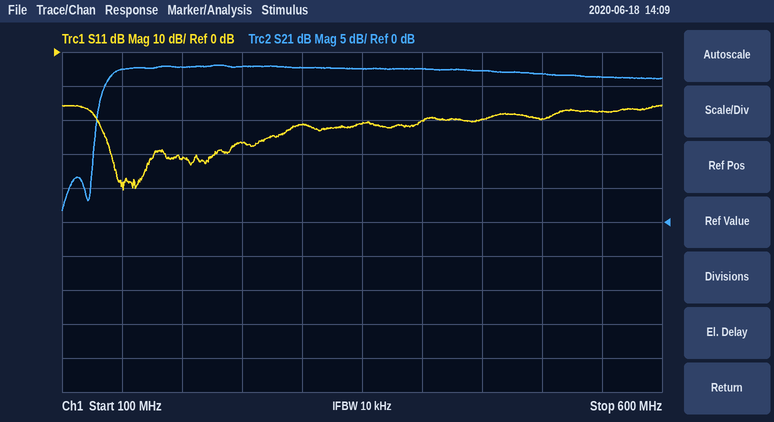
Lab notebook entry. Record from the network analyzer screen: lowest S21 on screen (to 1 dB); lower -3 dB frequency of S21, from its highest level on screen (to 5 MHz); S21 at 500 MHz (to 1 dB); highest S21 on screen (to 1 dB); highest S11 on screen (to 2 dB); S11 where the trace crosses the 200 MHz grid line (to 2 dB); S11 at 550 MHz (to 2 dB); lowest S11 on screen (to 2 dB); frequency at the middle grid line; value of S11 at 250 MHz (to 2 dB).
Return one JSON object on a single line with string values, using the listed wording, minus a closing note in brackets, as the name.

{"lowest S21 on screen": "2 dB", "lower -3 dB frequency of S21, from its highest level on screen": "135 MHz", "S21 at 500 MHz": "22 dB", "highest S21 on screen": "23 dB", "highest S11 on screen": "-16 dB", "S11 where the trace crosses the 200 MHz grid line": "-32 dB", "S11 at 550 MHz": "-18 dB", "lowest S11 on screen": "-40 dB", "frequency at the middle grid line": "350 MHz", "value of S11 at 250 MHz": "-26 dB"}
